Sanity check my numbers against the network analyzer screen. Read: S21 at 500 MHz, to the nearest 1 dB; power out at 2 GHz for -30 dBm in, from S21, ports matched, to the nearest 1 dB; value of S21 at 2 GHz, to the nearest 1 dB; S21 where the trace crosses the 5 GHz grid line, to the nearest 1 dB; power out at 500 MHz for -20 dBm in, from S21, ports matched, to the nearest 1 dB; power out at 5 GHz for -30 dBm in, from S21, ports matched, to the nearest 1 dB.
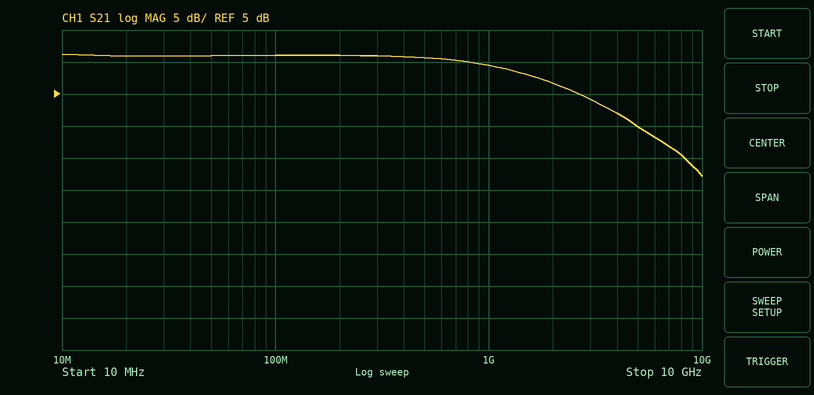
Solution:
11 dB
-23 dBm
7 dB
0 dB
-9 dBm
-30 dBm
